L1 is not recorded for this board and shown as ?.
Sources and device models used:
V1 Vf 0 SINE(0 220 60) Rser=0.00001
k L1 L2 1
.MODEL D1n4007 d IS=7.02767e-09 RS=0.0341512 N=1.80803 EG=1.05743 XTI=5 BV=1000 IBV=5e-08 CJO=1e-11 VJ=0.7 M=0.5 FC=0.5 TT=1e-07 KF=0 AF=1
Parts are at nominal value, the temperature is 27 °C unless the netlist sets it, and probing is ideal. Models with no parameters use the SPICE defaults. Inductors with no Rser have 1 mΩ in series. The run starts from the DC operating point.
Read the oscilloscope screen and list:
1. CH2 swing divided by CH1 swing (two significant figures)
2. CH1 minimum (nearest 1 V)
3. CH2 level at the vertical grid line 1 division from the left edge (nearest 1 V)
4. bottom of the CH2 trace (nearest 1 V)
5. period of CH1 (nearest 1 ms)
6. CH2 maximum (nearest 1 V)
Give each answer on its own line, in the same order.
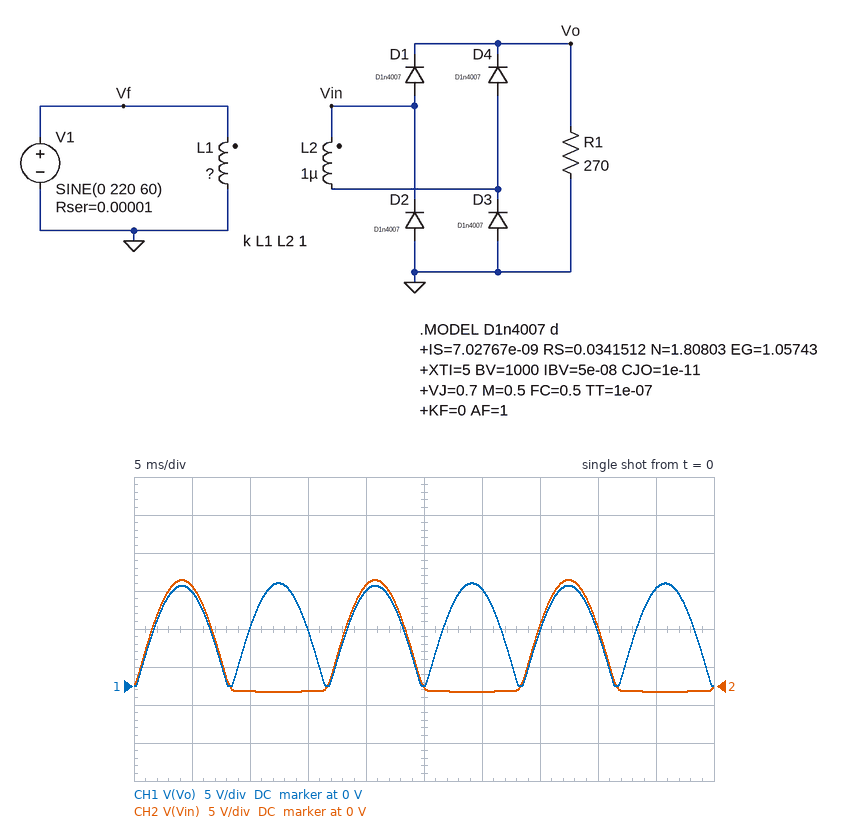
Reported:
1.1
0 V
13 V
-1 V
8 ms
14 V
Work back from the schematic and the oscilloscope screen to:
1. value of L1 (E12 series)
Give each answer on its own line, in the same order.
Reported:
220 µH
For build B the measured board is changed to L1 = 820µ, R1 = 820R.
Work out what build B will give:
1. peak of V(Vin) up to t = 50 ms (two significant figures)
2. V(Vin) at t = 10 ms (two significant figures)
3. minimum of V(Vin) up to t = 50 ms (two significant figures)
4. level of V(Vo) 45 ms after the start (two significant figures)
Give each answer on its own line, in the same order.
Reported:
7.0 V
-620 mV
-650 mV
6.0 V
